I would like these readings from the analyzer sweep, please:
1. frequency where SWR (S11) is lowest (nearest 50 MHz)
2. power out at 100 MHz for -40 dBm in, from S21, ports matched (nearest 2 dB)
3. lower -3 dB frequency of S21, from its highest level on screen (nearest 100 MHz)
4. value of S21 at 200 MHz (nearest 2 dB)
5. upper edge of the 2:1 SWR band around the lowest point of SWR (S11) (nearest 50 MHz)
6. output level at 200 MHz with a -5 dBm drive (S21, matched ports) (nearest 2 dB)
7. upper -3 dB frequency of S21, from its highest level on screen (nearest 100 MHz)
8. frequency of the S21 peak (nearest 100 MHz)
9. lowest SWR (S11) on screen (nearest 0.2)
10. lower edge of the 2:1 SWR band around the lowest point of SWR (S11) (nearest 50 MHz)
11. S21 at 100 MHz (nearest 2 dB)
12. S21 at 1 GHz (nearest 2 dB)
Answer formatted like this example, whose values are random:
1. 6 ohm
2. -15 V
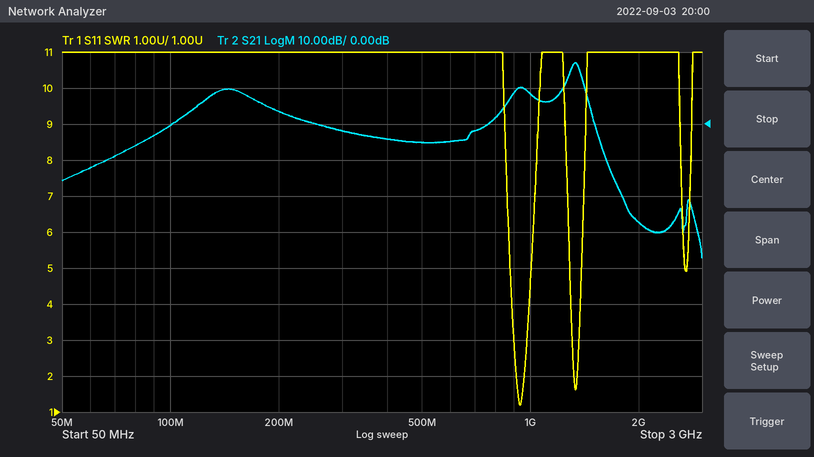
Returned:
1. 950 MHz
2. -40 dBm
3. 1.3 GHz
4. 4 dB
5. 950 MHz
6. -2 dBm
7. 1.4 GHz
8. 1.3 GHz
9. 1.2
10. 900 MHz
11. 0 dB
12. 8 dB
